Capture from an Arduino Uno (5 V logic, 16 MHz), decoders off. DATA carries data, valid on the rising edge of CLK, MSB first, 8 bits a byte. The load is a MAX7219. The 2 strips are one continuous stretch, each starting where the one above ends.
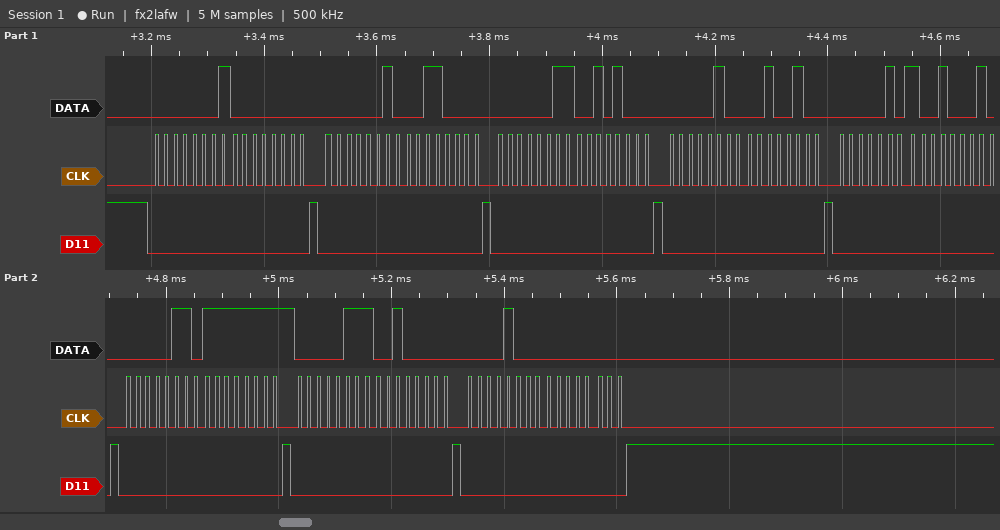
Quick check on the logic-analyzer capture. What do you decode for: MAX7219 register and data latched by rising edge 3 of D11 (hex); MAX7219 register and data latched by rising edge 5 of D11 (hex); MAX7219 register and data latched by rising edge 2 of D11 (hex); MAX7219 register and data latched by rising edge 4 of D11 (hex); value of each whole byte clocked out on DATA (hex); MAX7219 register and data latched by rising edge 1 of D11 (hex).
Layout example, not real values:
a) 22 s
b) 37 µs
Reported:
a) register 0x3, data 0x28
b) register 0x5, data 0x22
c) register 0x2, data 0x30
d) register 0x4, data 0x24
e) 0x01 0x00 0x02 0x30 0x03 0x28 0x04 0x24 0x05 0x22 0x06 0xFF 0x07 0x20 0x08 0x00
f) register 0x1, data 0x00
